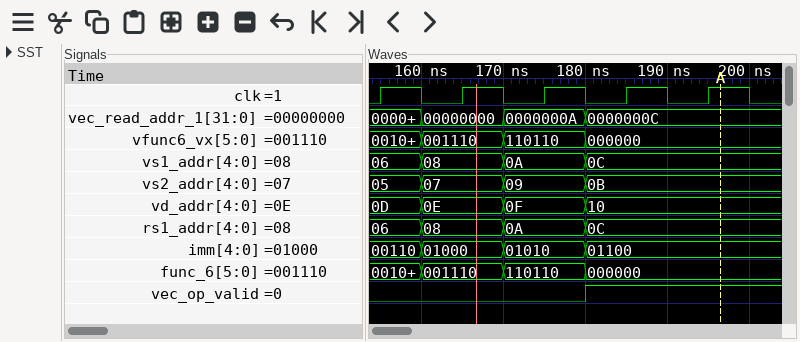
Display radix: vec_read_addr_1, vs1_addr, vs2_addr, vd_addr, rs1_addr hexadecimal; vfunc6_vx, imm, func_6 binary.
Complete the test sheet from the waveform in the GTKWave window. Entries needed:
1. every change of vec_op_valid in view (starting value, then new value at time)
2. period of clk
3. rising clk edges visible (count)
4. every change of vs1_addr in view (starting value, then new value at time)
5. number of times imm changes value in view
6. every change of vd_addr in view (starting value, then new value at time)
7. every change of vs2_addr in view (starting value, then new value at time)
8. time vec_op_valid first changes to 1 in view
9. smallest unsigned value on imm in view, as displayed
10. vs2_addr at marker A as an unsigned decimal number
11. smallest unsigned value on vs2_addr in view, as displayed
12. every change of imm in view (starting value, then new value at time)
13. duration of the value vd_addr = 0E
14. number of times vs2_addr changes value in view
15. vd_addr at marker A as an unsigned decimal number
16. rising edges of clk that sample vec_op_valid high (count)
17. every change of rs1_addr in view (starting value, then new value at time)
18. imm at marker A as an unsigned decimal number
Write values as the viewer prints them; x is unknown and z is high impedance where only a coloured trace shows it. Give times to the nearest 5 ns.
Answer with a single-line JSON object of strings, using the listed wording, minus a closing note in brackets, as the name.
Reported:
{"every change of vec_op_valid in view": "0, 1 at 180 ns", "period of clk": "10 ns", "rising clk edges visible": "5", "every change of vs1_addr in view": "06, 08 at 160 ns, 0A at 170 ns, 0C at 180 ns", "number of times imm changes value in view": "3", "every change of vd_addr in view": "0D, 0E at 160 ns, 0F at 170 ns, 10 at 180 ns", "every change of vs2_addr in view": "05, 07 at 160 ns, 09 at 170 ns, 0B at 180 ns", "time vec_op_valid first changes to 1 in view": "180 ns", "smallest unsigned value on imm in view, as displayed": "00110", "vs2_addr at marker A as an unsigned decimal number": "11", "smallest unsigned value on vs2_addr in view, as displayed": "05", "every change of imm in view": "00110, 01000 at 160 ns, 01010 at 170 ns, 01100 at 180 ns", "duration of the value vd_addr = 0E": "10 ns", "number of times vs2_addr changes value in view": "3", "vd_addr at marker A as an unsigned decimal number": "16", "rising edges of clk that sample vec_op_valid high": "2", "every change of rs1_addr in view": "06, 08 at 160 ns, 0A at 170 ns, 0C at 180 ns", "imm at marker A as an unsigned decimal number": "12"}
